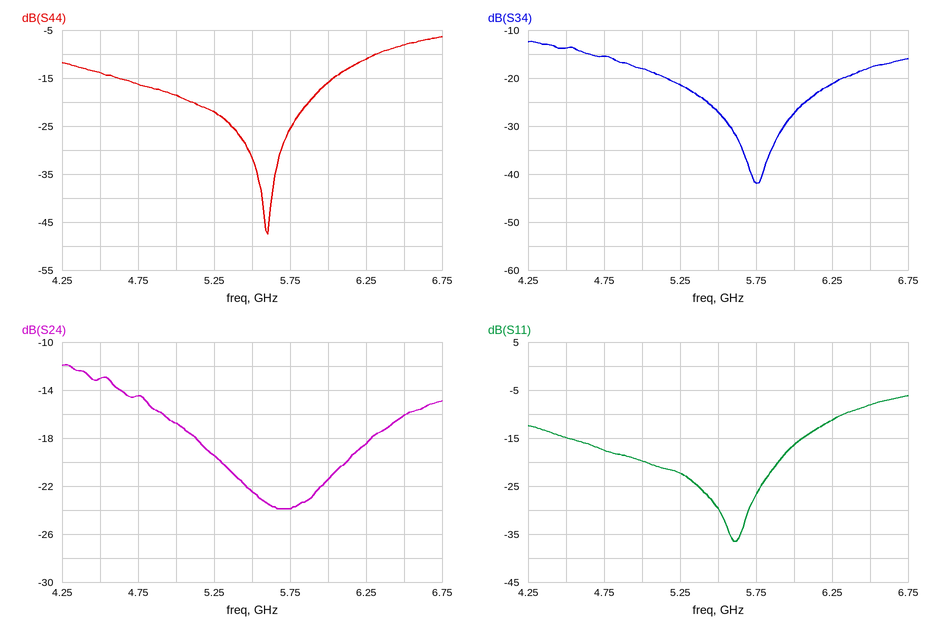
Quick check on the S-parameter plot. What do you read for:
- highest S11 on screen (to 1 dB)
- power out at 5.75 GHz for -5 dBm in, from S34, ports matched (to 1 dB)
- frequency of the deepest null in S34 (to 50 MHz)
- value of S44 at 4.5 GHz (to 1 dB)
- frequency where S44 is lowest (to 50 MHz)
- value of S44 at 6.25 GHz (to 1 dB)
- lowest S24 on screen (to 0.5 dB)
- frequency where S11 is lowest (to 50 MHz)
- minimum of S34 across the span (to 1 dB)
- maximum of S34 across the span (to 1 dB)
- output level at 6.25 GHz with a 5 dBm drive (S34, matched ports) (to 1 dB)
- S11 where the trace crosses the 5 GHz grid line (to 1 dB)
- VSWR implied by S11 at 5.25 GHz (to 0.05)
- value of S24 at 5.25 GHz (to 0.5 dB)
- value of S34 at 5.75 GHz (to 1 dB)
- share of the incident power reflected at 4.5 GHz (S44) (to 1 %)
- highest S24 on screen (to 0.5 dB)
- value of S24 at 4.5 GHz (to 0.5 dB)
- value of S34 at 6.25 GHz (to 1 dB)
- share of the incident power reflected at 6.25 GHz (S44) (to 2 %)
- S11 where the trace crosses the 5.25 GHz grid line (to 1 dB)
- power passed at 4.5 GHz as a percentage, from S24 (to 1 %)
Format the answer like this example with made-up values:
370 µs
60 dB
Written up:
-6 dB
-47 dBm
5.75 GHz
-14 dB
5.60 GHz
-11 dB
-24.0 dB
5.60 GHz
-42 dB
-12 dB
-16 dBm
-20 dB
1.15
-19.5 dB
-42 dB
4 %
-12.0 dB
-13.0 dB
-21 dB
8 %
-22 dB
5 %
